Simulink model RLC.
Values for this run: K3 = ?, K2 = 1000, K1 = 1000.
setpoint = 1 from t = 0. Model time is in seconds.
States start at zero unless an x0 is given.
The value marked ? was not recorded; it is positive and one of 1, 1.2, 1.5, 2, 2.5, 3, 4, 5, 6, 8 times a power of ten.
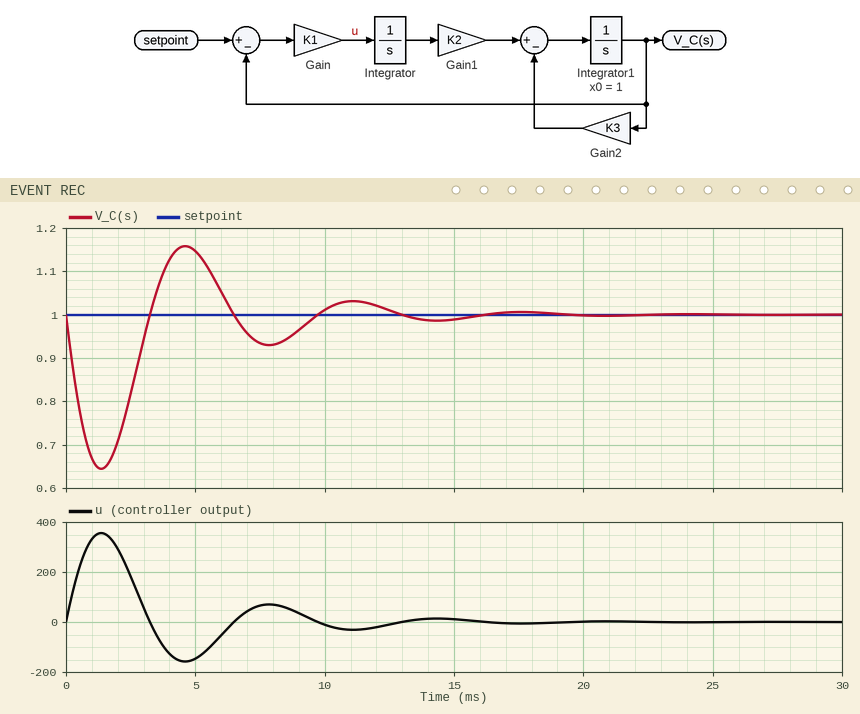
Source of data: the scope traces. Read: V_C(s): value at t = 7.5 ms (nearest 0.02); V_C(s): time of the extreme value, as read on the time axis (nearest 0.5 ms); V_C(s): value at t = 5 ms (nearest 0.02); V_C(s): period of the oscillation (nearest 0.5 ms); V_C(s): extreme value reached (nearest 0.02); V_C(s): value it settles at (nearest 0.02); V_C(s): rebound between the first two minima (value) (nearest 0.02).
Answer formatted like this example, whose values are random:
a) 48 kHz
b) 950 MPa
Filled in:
a) 0.94
b) 1.5 ms
c) 1.14
d) 6.5 ms
e) 0.64
f) 1.00
g) 1.16
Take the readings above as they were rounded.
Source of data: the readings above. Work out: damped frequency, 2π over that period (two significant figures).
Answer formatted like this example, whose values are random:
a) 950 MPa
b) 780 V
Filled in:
a) 0.97 rad/ms
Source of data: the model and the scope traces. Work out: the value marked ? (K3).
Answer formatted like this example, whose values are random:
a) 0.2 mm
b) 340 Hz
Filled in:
a) 500
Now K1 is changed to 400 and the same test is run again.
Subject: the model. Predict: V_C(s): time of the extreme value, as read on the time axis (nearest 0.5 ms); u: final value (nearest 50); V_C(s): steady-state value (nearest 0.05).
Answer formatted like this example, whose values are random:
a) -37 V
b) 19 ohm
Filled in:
a) 2.0 ms
b) 0
c) 1.00
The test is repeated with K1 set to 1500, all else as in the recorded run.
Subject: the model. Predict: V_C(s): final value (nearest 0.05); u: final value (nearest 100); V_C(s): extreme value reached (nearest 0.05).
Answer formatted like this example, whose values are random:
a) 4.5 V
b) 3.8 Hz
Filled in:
a) 1.00
b) 0
c) 0.70
